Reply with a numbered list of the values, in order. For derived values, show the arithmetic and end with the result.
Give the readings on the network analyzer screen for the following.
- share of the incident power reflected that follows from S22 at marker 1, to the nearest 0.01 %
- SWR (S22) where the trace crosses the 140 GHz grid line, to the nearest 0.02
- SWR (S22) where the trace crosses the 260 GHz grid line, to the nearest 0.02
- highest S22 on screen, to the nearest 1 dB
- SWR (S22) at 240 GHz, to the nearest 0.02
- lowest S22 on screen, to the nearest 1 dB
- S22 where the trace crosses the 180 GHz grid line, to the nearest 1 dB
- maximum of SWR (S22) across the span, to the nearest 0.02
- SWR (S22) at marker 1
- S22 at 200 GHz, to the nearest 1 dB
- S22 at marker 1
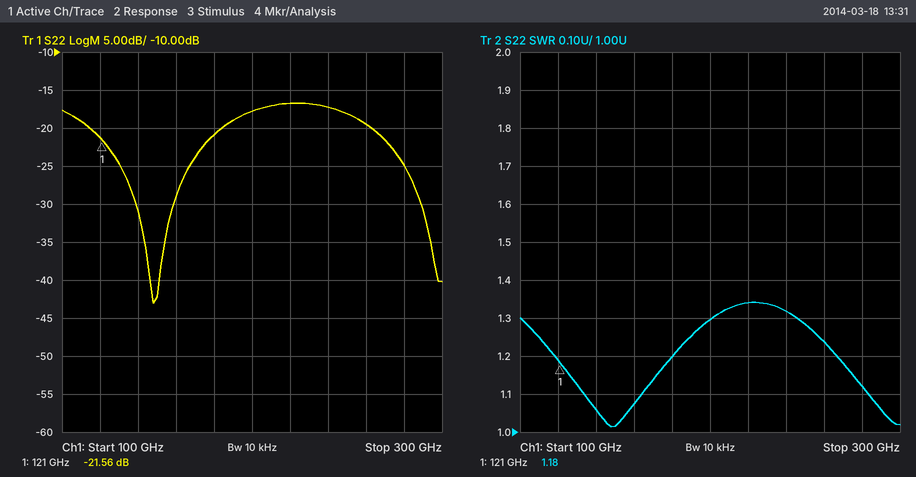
1. 10^(-21.56/10) ≈ 0.70 %
2. 1.06
3. 1.24
4. -17 dB
5. 1.32
6. -43 dB
7. -21 dB
8. 1.34
9. 1.18
10. -18 dB
11. -21.56 dB
